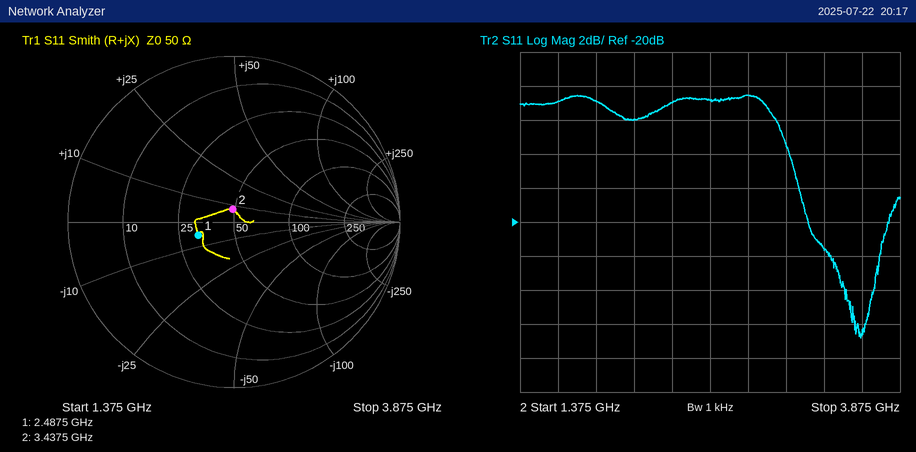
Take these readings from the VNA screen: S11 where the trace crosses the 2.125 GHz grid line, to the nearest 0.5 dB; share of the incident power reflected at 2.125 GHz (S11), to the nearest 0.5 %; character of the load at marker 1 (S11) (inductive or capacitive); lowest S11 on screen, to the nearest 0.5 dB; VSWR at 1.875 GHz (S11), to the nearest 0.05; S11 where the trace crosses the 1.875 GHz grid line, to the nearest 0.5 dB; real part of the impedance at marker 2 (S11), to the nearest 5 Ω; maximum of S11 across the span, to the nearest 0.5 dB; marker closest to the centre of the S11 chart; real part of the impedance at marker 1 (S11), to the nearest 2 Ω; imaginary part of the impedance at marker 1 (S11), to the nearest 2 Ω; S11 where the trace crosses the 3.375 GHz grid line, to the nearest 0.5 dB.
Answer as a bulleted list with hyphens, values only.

- -14.0 dB
- 4.0 %
- capacitive
- -27.0 dB
- 1.60
- -13.0 dB
- 50 Ω
- -12.5 dB
- marker 2
- 32 Ω
- -6 Ω
- -21.5 dB
